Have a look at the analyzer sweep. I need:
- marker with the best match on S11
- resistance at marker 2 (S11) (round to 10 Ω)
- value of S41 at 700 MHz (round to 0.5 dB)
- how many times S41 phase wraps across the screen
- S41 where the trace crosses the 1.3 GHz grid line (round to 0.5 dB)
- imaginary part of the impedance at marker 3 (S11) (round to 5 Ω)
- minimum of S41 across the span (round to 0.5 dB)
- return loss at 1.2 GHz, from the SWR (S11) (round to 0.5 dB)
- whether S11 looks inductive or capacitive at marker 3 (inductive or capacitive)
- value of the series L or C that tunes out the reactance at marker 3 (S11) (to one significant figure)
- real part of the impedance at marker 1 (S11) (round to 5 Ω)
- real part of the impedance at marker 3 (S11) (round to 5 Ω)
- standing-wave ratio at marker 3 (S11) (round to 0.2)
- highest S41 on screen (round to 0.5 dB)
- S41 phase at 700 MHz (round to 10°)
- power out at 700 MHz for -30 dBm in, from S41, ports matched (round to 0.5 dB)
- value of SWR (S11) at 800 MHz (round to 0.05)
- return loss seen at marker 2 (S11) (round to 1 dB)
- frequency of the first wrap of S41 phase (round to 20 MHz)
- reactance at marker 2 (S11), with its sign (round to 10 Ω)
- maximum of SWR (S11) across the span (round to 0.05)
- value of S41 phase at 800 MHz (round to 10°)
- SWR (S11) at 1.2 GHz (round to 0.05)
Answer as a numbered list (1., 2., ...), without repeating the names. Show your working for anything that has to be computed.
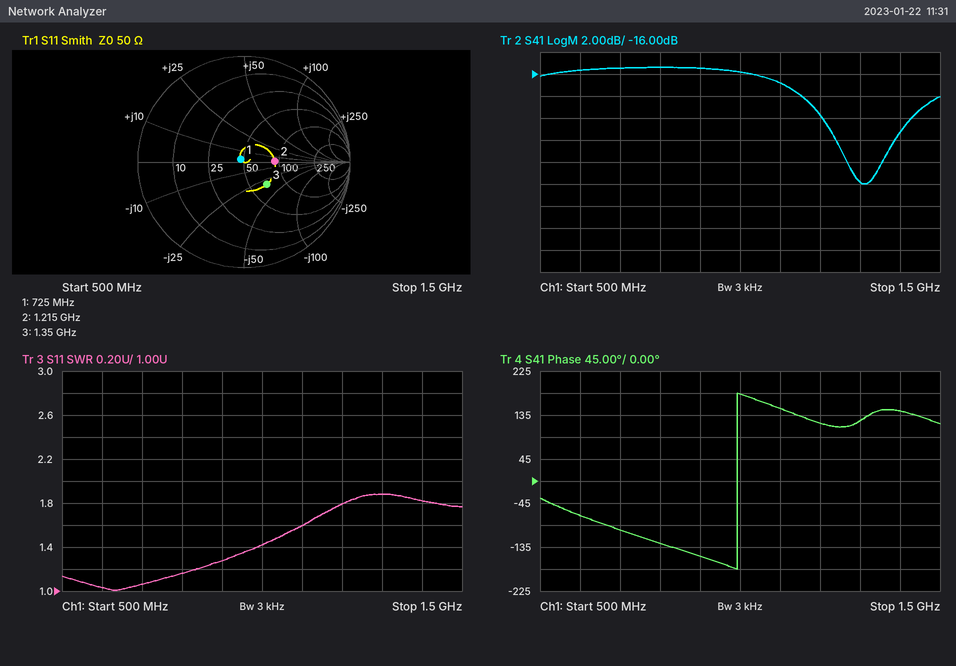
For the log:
1. marker 1
2. 90 Ω
3. -15.5 dB
4. 1
5. -26.0 dB
6. -30 Ω
7. -26.0 dB
8. −20 log10((1.8 − 1)/(1.8 + 1)) ≈ 10.9 dB, so 11.0 dB to the nearest 0.5 dB
9. capacitive
10. L = 30 Ω/(2π × 1.35 GHz) ≈ 4 nH
11. 45 Ω
12. 70 Ω
13. 1.8
14. -15.5 dB
15. -100°
16. -30 dBm + (-15.5 dB) = -45.5 dBm
17. 1.15
18. 11 dB
19. 1.00 GHz
20. 0 Ω
21. 1.90
22. -130°
23. 1.80
